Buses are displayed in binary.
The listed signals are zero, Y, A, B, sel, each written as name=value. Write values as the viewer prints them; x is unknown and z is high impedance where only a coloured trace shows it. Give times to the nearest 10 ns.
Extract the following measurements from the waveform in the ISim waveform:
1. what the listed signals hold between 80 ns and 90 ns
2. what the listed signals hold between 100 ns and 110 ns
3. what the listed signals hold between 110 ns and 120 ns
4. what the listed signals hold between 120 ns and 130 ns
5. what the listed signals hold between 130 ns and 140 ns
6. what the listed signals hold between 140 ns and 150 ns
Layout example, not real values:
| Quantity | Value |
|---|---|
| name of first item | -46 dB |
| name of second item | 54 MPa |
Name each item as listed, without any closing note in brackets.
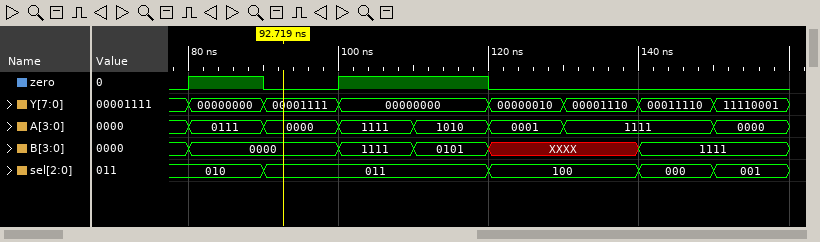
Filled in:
| Quantity | Value |
|---|---|
| what the listed signals hold between 80 ns and 90 ns | zero=1, Y=00000000, A=0111, B=0000, sel=010 |
| what the listed signals hold between 100 ns and 110 ns | zero=1, Y=00000000, A=1111, B=1111, sel=011 |
| what the listed signals hold between 110 ns and 120 ns | zero=1, Y=00000000, A=1010, B=0101, sel=011 |
| what the listed signals hold between 120 ns and 130 ns | zero=0, Y=00000010, A=0001, B=XXXX, sel=100 |
| what the listed signals hold between 130 ns and 140 ns | zero=0, Y=00001110, A=1111, B=XXXX, sel=100 |
| what the listed signals hold between 140 ns and 150 ns | zero=0, Y=00011110, A=1111, B=1111, sel=000 |
